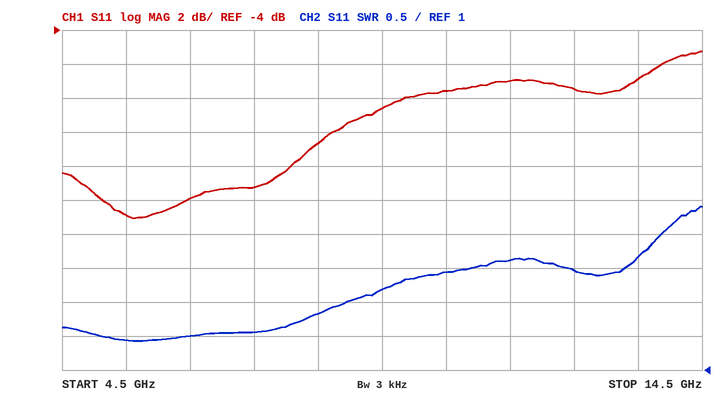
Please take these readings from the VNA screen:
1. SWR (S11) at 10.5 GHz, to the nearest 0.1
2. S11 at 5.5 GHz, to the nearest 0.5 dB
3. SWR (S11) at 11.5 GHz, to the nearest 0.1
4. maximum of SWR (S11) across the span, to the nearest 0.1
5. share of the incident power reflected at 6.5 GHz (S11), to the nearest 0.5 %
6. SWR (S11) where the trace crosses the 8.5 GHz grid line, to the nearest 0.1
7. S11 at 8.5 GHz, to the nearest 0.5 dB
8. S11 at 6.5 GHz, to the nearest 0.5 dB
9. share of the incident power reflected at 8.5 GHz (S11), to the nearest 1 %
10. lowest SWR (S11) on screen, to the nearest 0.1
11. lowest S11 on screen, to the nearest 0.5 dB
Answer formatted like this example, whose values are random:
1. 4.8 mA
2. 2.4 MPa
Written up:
1. 2.4
2. -15.0 dB
3. 2.6
4. 3.4
5. 4.0 %
6. 1.8
7. -10.5 dB
8. -14.0 dB
9. 9 %
10. 1.4
11. -15.0 dB
